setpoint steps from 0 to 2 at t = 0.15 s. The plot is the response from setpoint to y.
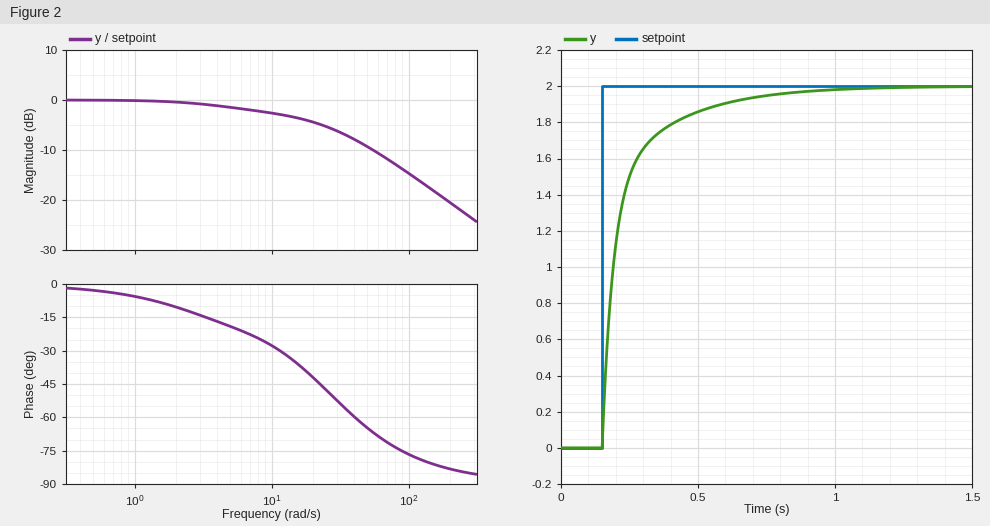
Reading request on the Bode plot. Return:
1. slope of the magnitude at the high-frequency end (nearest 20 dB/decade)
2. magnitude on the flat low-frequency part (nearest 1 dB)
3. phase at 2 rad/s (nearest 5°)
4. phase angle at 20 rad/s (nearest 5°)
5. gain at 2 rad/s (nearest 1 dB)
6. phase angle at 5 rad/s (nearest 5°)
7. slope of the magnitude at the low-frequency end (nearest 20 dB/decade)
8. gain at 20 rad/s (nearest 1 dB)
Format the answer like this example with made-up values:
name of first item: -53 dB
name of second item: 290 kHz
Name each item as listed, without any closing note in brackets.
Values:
slope of the magnitude at the high-frequency end: -20 dB/decade
magnitude on the flat low-frequency part: 0 dB
phase at 2 rad/s: -10°
phase angle at 20 rad/s: -40°
gain at 2 rad/s: 0 dB
phase angle at 5 rad/s: -20°
slope of the magnitude at the low-frequency end: 0 dB/decade
gain at 20 rad/s: -4 dB
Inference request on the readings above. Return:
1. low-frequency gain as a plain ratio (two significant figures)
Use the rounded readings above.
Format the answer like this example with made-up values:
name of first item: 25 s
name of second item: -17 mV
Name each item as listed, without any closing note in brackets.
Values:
low-frequency gain as a plain ratio: 1.0
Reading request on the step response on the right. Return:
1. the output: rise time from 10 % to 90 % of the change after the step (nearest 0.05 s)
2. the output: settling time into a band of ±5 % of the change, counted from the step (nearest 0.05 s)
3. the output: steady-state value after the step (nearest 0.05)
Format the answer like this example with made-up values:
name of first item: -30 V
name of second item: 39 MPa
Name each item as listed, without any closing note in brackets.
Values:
the output: rise time from 10 % to 90 % of the change after the step: 0.25 s
the output: settling time into a band of ±5 % of the change, counted from the step: 0.45 s
the output: steady-state value after the step: 2.00
